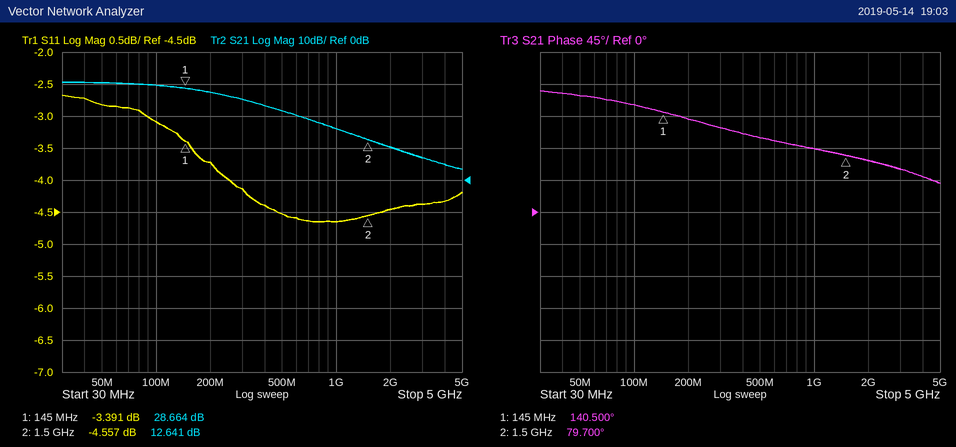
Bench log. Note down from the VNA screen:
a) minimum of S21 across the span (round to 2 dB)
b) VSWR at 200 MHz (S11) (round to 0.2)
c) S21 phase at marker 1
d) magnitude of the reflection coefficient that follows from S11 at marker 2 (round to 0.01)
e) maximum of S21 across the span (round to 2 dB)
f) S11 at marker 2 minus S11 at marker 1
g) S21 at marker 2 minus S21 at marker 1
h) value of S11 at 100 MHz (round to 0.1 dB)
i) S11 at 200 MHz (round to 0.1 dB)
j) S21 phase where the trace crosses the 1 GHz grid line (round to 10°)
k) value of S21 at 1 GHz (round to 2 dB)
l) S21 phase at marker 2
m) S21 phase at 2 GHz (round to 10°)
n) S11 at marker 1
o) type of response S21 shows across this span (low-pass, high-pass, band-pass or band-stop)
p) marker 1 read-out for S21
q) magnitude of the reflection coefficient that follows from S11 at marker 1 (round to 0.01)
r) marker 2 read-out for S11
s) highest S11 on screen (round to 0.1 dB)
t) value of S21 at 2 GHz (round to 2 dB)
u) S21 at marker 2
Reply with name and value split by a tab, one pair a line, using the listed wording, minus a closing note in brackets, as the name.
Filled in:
minimum of S21 across the span	4 dB
VSWR at 200 MHz (S11)	4.8
S21 phase at marker 1	140.500°
magnitude of the reflection coefficient that follows from S11 at marker 2	0.59
maximum of S21 across the span	30 dB
S11 at marker 2 minus S11 at marker 1	-1.166 dB
S21 at marker 2 minus S21 at marker 1	-16.023 dB
value of S11 at 100 MHz	-3.1 dB
S11 at 200 MHz	-3.7 dB
S21 phase where the trace crosses the 1 GHz grid line	90°
value of S21 at 1 GHz	16 dB
S21 phase at marker 2	79.700°
S21 phase at 2 GHz	70°
S11 at marker 1	-3.391 dB
type of response S21 shows across this span	low-pass
marker 1 read-out for S21	28.664 dB
magnitude of the reflection coefficient that follows from S11 at marker 1	0.68
marker 2 read-out for S11	-4.557 dB
highest S11 on screen	-2.7 dB
value of S21 at 2 GHz	10 dB
S21 at marker 2	12.641 dB
